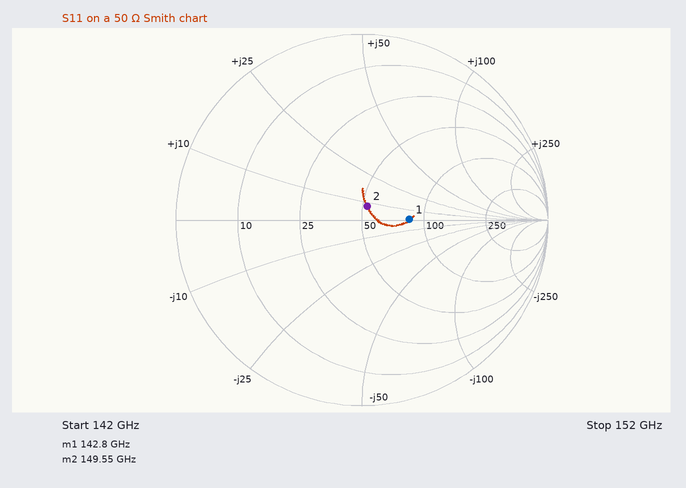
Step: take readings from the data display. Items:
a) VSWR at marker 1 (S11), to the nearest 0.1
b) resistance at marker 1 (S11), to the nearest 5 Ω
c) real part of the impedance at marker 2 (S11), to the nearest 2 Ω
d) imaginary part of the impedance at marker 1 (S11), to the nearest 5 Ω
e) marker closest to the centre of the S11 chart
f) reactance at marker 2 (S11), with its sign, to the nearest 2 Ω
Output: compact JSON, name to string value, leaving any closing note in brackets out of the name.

{"VSWR at marker 1 (S11), to the nearest 0.1": "1.7", "resistance at marker 1 (S11), to the nearest 5 Ω": "85 Ω", "real part of the impedance at marker 2 (S11), to the nearest 2 Ω": "52 Ω", "imaginary part of the impedance at marker 1 (S11), to the nearest 5 Ω": "0 Ω", "marker closest to the centre of the S11 chart": "marker 2", "reactance at marker 2 (S11), with its sign, to the nearest 2 Ω": "+8 Ω"}
